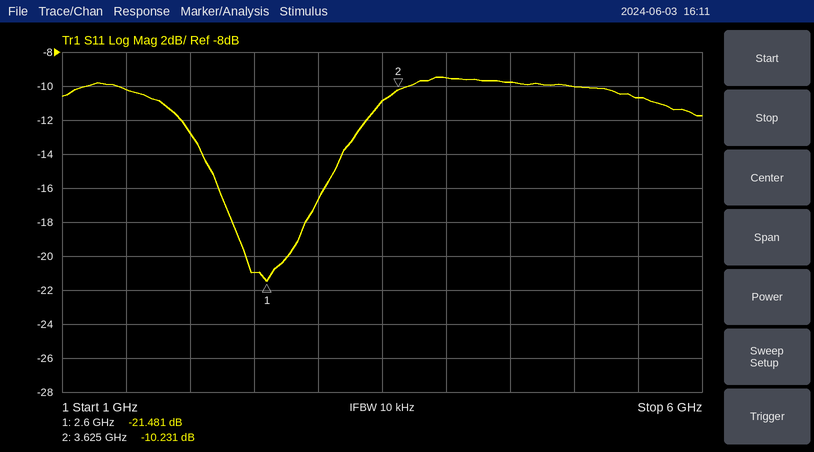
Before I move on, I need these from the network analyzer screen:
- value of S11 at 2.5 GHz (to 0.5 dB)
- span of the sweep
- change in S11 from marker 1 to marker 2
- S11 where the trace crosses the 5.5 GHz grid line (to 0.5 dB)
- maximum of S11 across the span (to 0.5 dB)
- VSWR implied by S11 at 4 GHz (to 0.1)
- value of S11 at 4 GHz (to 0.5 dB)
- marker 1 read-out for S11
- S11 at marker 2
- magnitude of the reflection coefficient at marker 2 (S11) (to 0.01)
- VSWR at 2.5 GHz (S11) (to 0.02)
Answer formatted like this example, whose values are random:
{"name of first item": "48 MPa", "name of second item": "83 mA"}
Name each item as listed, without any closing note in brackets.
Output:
{"value of S11 at 2.5 GHz": "-21.0 dB", "span of the sweep": "5 GHz", "change in S11 from marker 1 to marker 2": "11.250 dB", "S11 where the trace crosses the 5.5 GHz grid line": "-10.5 dB", "maximum of S11 across the span": "-9.5 dB", "VSWR implied by S11 at 4 GHz": "2.0", "value of S11 at 4 GHz": "-9.5 dB", "marker 1 read-out for S11": "-21.481 dB", "S11 at marker 2": "-10.231 dB", "magnitude of the reflection coefficient at marker 2 (S11)": "0.31", "VSWR at 2.5 GHz (S11)": "1.20"}
